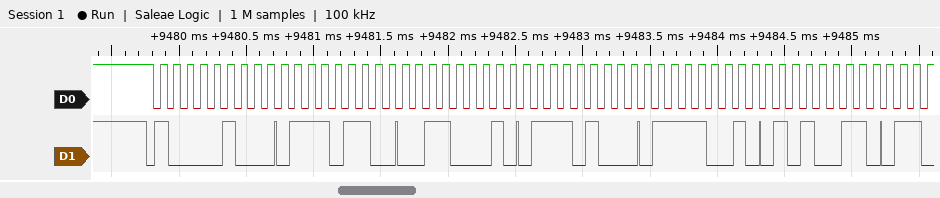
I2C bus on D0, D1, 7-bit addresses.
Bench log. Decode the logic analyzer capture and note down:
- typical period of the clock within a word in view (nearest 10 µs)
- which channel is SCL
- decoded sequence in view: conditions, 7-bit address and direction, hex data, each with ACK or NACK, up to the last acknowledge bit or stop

100 µs
D0
start, address 42 write ACK, 76 ACK, 31 ACK, 74 ACK, 79 ACK, 53 ACK
